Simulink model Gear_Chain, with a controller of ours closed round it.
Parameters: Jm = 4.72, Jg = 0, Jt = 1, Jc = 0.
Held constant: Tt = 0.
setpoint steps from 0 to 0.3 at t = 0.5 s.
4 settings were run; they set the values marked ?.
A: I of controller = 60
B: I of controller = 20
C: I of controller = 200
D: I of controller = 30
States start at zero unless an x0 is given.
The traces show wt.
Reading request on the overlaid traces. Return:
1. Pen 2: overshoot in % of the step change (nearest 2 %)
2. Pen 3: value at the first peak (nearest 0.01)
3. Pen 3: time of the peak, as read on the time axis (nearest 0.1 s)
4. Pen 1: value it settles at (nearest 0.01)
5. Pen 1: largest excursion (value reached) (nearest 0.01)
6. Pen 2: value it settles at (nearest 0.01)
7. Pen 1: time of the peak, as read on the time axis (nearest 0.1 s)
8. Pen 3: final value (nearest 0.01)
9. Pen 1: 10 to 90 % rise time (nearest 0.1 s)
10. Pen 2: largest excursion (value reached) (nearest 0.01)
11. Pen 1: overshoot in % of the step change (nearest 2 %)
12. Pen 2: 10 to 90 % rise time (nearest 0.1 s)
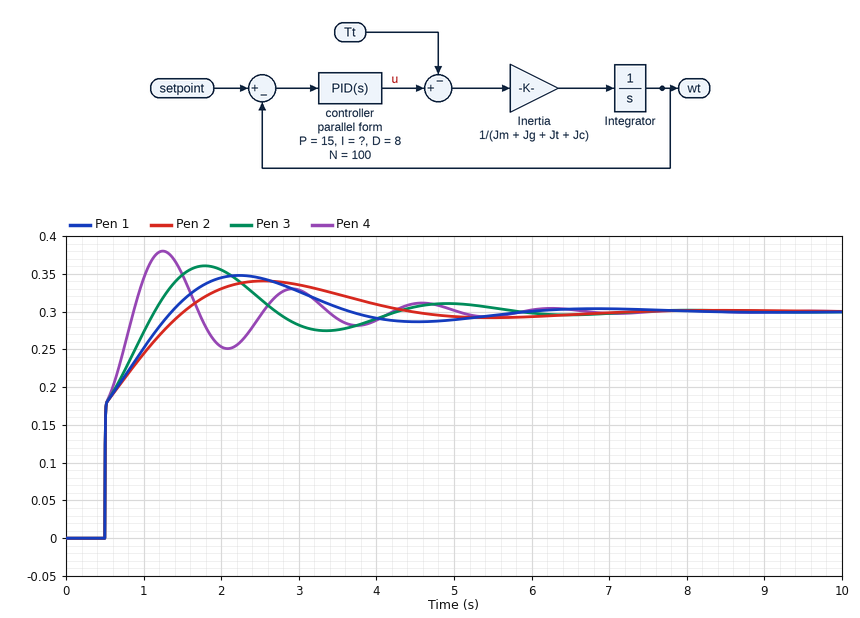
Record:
14 %
0.36
1.8 s
0.30
0.35
0.30
2.2 s
0.30
0.6 s
0.34
16 %
0.7 s
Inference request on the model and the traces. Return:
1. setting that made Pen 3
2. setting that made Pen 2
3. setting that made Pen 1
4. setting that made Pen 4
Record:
A
B
D
C
